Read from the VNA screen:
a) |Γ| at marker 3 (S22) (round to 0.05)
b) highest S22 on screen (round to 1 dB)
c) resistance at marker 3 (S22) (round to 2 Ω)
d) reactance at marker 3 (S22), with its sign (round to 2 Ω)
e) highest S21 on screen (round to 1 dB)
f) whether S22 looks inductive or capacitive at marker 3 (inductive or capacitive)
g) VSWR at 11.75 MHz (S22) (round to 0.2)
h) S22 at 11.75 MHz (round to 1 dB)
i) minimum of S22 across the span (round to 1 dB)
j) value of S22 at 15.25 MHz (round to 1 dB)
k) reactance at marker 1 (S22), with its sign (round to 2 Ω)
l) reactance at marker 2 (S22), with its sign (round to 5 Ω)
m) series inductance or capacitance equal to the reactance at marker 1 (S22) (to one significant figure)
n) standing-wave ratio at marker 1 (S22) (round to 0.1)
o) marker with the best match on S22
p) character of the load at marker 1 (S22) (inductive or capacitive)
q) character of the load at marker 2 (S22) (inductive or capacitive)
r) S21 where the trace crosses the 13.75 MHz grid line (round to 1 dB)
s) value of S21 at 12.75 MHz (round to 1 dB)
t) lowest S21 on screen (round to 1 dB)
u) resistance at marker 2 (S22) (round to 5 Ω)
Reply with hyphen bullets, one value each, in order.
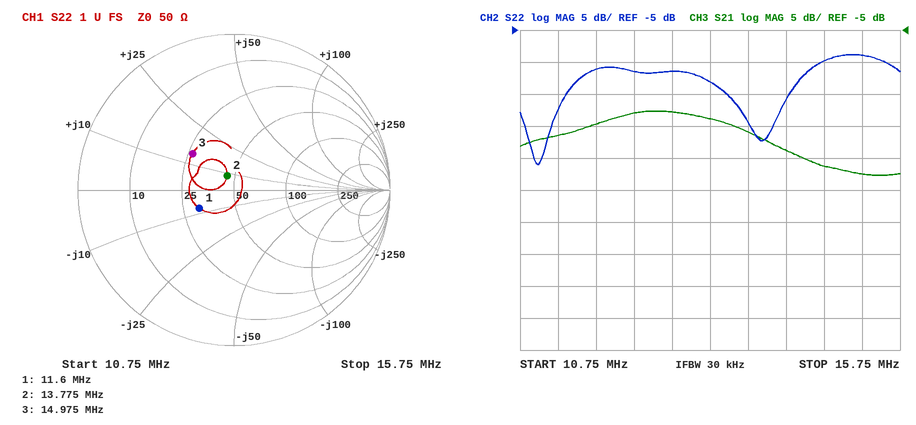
- 0.35
- -9 dB
- 26 Ω
- +14 Ω
- -18 dB
- inductive
- 1.8
- -11 dB
- -26 dB
- -9 dB
- -8 Ω
- +10 Ω
- 2 nF
- 1.7
- marker 2
- capacitive
- inductive
- -21 dB
- -18 dB
- -28 dB
- 45 Ω
